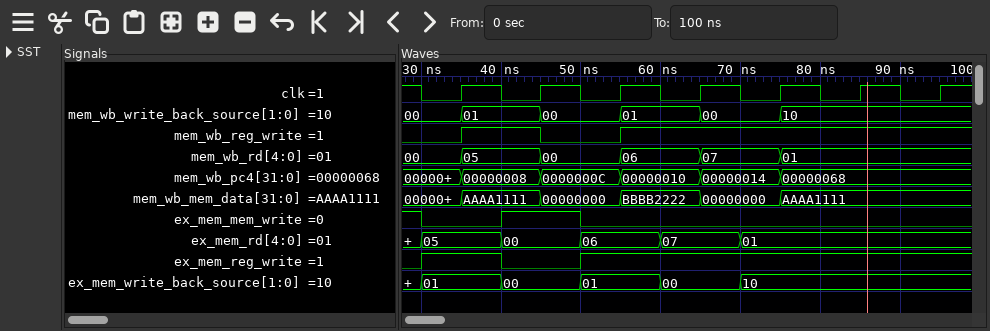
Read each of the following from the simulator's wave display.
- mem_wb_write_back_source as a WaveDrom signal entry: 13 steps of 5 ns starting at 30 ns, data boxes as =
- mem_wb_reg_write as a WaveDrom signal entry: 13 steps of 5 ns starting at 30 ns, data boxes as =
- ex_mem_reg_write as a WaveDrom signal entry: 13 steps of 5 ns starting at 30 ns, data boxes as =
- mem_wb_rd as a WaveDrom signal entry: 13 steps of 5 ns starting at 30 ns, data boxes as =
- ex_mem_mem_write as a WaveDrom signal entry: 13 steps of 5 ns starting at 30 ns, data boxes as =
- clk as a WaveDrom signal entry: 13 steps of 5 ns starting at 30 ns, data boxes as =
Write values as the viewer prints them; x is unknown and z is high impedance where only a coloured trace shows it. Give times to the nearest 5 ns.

{name: 'mem_wb_write_back_source', wave: '==.=.=.=.=...', data: '00 01 00 01 00 10'}
{name: 'mem_wb_reg_write', wave: '01.0.1.......'}
{name: 'ex_mem_reg_write', wave: '1.0.1........'}
{name: 'mem_wb_rd', wave: '==.=.=.=.=...', data: '00 05 00 06 07 01'}
{name: 'ex_mem_mem_write', wave: '0.1.0........'}
{name: 'clk', wave: '0101010101010'}
